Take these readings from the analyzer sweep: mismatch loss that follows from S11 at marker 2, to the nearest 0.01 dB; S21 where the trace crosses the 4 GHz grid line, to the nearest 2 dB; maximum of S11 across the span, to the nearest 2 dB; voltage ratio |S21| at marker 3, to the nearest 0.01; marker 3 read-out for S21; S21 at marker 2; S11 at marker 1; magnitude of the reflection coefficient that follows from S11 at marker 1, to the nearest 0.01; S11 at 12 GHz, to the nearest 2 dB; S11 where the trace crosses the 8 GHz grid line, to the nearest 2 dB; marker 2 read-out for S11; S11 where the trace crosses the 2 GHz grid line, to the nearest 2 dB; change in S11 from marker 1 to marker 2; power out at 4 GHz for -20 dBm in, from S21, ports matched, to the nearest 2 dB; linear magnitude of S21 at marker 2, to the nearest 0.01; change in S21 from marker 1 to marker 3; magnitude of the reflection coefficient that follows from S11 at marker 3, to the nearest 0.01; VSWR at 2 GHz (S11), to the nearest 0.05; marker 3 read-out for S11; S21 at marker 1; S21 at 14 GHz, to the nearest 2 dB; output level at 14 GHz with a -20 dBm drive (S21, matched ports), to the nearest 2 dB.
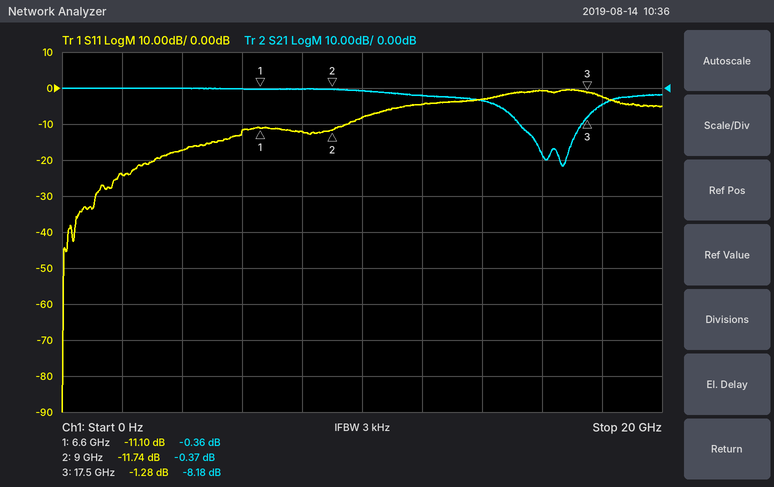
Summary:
0.30 dB
0 dB
0 dB
0.39
-8.18 dB
-0.37 dB
-11.10 dB
0.28
-4 dB
-12 dB
-11.74 dB
-24 dB
-0.64 dB
-20 dBm
0.96
-7.82 dB
0.86
1.15
-1.28 dB
-0.36 dB
-4 dB
-24 dBm
